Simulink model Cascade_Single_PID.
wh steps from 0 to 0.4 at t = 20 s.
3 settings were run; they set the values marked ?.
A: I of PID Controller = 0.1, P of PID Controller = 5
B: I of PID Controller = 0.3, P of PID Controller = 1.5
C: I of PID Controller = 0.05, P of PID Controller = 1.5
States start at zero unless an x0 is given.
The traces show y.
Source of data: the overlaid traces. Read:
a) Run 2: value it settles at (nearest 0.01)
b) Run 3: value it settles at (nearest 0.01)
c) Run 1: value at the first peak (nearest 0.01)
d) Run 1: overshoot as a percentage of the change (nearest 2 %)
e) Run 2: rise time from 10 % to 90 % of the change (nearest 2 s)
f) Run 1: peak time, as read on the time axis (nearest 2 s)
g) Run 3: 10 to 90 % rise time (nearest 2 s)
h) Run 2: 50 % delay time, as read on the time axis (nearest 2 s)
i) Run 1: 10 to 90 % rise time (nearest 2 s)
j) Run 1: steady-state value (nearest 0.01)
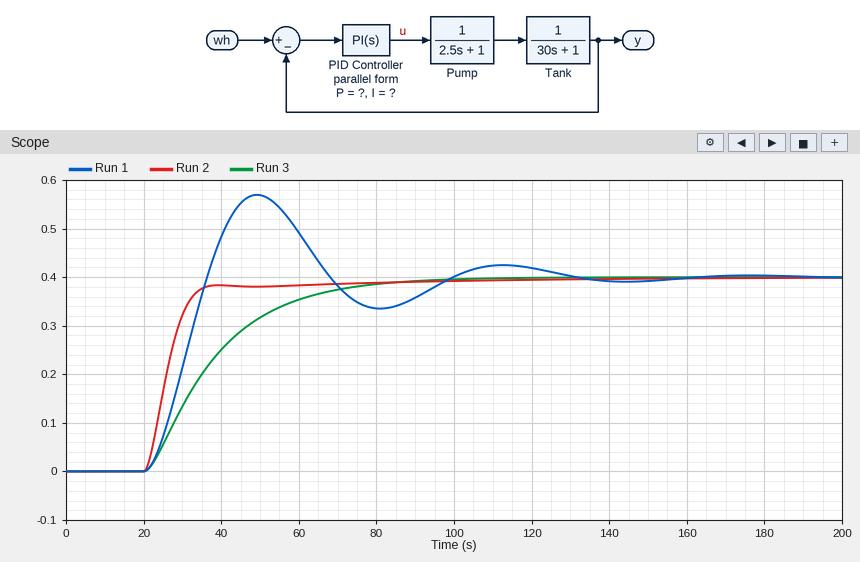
0.40
0.40
0.57
42 %
10 s
50 s
38 s
26 s
12 s
0.40
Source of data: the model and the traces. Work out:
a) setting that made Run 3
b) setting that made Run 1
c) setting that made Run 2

C
B
A
